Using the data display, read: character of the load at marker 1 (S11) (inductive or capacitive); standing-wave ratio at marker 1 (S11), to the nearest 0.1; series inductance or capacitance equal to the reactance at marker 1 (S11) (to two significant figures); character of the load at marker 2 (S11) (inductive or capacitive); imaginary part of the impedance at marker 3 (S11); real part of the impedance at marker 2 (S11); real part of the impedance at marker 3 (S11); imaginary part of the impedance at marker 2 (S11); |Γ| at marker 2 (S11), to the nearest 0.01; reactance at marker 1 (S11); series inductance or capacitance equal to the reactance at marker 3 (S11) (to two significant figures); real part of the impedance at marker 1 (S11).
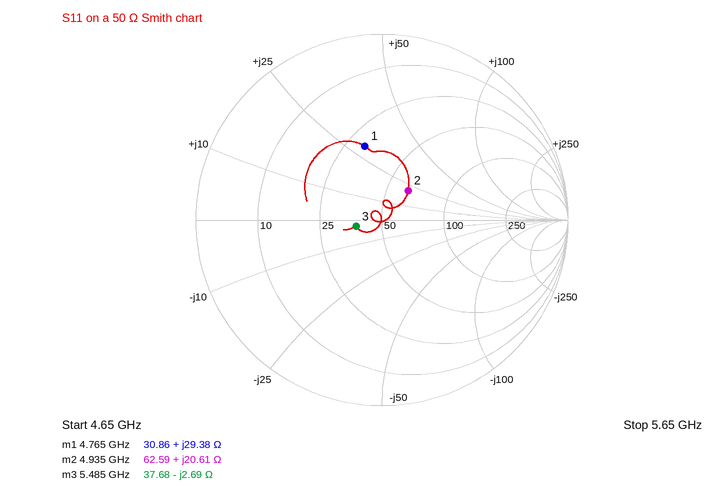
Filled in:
inductive
2.4
980 pH
inductive
-2.69 Ω
62.59 Ω
37.68 Ω
+20.61 Ω
0.21
+29.38 Ω
11 pF
30.86 Ω
